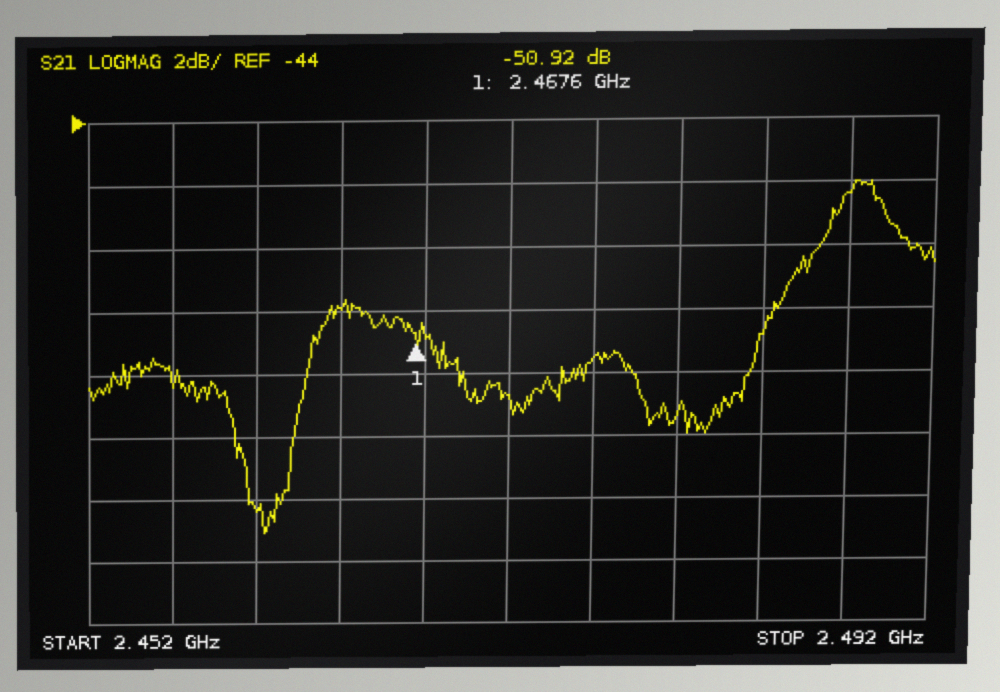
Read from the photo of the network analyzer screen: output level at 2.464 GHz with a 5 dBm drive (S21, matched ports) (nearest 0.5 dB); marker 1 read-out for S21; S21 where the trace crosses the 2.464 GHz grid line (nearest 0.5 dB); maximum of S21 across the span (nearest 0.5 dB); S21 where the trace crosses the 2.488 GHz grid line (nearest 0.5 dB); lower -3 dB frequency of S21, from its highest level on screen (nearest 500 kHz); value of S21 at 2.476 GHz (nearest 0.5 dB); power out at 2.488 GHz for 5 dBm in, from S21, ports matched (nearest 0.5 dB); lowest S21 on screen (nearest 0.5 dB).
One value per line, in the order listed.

-45.0 dBm
-50.92 dB
-50.0 dB
-46.0 dB
-46.5 dB
2.4855 GHz
-51.5 dB
-41.5 dBm
-57.0 dB
